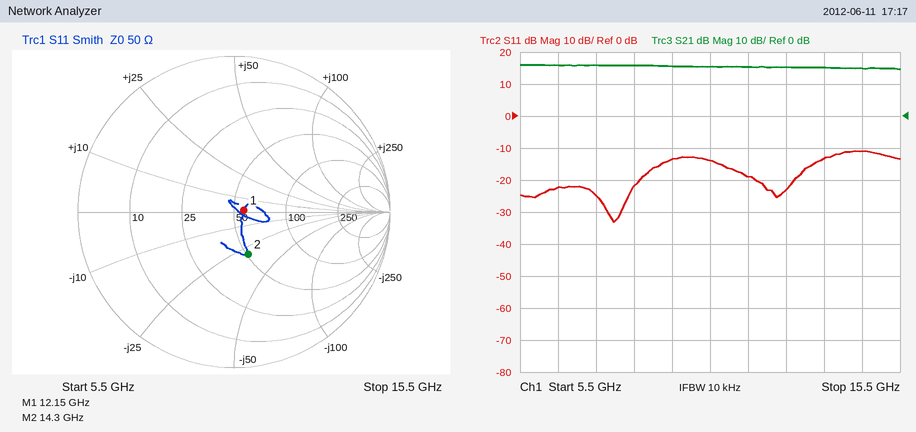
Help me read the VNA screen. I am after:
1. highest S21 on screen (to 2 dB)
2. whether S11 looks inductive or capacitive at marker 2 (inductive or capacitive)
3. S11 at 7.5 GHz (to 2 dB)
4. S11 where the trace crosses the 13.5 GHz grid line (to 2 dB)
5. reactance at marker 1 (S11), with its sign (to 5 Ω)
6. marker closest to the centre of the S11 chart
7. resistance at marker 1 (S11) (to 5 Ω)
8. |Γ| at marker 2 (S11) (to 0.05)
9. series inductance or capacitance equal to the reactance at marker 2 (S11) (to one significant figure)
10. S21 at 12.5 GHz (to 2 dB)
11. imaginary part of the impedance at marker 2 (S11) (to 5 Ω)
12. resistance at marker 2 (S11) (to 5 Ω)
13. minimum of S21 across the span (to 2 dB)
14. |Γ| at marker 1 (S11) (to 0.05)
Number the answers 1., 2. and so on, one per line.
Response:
1. 16 dB
2. capacitive
3. -24 dB
4. -14 dB
5. 0 Ω
6. marker 1
7. 55 Ω
8. 0.30
9. 400 fF
10. 16 dB
11. -30 Ω
12. 50 Ω
13. 14 dB
14. 0.05
